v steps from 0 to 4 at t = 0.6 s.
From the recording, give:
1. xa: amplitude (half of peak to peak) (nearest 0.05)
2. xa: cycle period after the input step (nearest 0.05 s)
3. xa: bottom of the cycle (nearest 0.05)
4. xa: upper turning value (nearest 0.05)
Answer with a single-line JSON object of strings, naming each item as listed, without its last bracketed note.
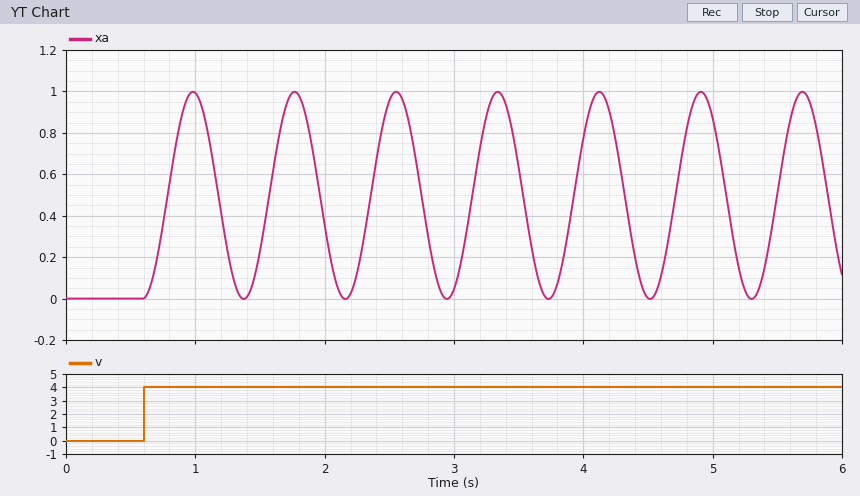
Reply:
{"xa: amplitude (half of peak to peak)": "0.50", "xa: cycle period after the input step": "0.80 s", "xa: bottom of the cycle": "0.00", "xa: upper turning value": "1.00"}
